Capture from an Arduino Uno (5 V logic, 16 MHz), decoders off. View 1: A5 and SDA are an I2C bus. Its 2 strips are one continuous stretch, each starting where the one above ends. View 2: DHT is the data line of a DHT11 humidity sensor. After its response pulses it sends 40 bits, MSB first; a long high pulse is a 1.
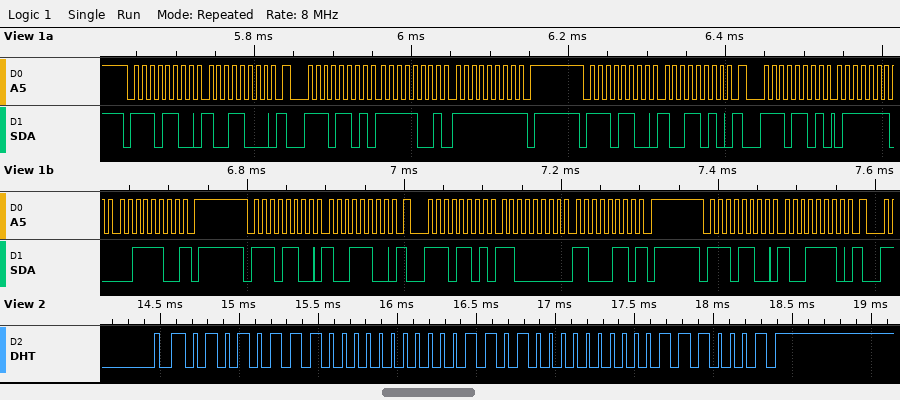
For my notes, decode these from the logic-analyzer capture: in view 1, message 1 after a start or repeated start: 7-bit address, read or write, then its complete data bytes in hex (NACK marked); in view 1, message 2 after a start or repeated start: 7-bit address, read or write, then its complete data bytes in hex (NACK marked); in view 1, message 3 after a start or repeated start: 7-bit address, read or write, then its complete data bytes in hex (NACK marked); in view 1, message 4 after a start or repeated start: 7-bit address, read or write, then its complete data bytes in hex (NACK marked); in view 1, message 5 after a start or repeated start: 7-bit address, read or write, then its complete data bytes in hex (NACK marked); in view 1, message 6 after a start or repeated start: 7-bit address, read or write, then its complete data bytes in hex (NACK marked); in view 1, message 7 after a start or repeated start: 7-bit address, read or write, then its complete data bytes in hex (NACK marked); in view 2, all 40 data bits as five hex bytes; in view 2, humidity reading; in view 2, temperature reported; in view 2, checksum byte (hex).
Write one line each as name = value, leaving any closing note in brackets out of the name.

in view 1, message 1 after a start or repeated start: 7-bit address, read or write, then its complete data bytes in hex = 0x76 write: 98
in view 1, message 2 after a start or repeated start: 7-bit address, read or write, then its complete data bytes in hex = 0x76 read: F9 FF NACK
in view 1, message 3 after a start or repeated start: 7-bit address, read or write, then its complete data bytes in hex = 0x76 write: 9A
in view 1, message 4 after a start or repeated start: 7-bit address, read or write, then its complete data bytes in hex = 0x76 read: 7E 3C NACK
in view 1, message 5 after a start or repeated start: 7-bit address, read or write, then its complete data bytes in hex = 0x76 write: 9C
in view 1, message 6 after a start or repeated start: 7-bit address, read or write, then its complete data bytes in hex = 0x76 read: C0 C6 NACK
in view 1, message 7 after a start or repeated start: 7-bit address, read or write, then its complete data bytes in hex = 0x76 write: 9E
in view 2, all 40 data bits as five hex bytes = 57 00 1A 00 71
in view 2, humidity reading = 87 %
in view 2, temperature reported = 26.0 °C
in view 2, checksum byte = 0x71
